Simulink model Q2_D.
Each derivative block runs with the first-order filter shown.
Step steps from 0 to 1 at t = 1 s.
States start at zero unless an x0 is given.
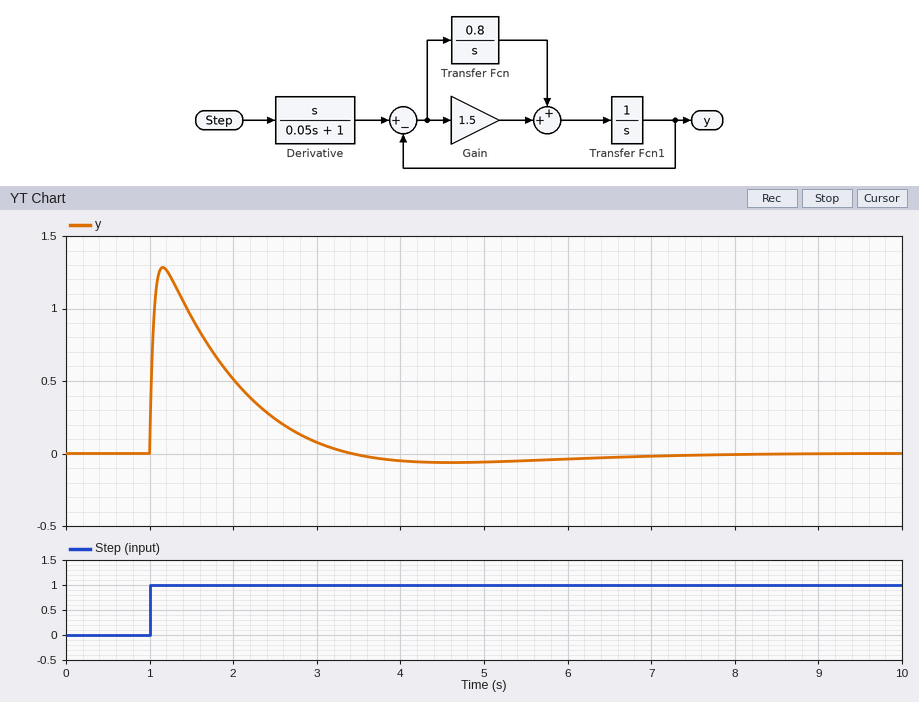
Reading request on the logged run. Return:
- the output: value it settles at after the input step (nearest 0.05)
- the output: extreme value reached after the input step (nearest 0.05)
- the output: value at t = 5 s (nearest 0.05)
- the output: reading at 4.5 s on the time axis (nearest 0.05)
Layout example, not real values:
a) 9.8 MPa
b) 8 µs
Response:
a) 0.00
b) 1.30
c) -0.05
d) -0.05
